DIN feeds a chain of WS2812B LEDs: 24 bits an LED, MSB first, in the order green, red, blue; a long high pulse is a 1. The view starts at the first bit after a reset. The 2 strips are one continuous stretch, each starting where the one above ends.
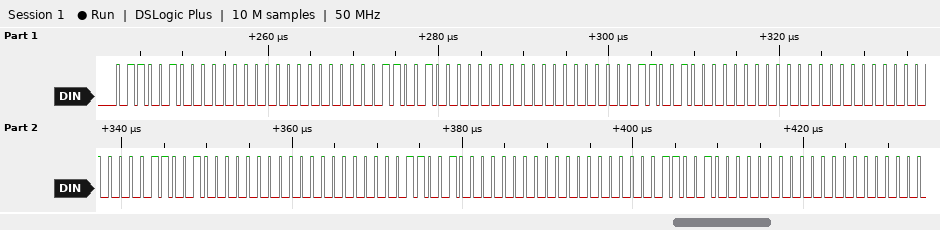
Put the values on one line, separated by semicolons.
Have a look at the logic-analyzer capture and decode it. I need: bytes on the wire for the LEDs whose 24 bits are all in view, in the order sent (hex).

64 00 00 64 00 00 64 00 00 00 64 00 00 64 00 00 64 00
